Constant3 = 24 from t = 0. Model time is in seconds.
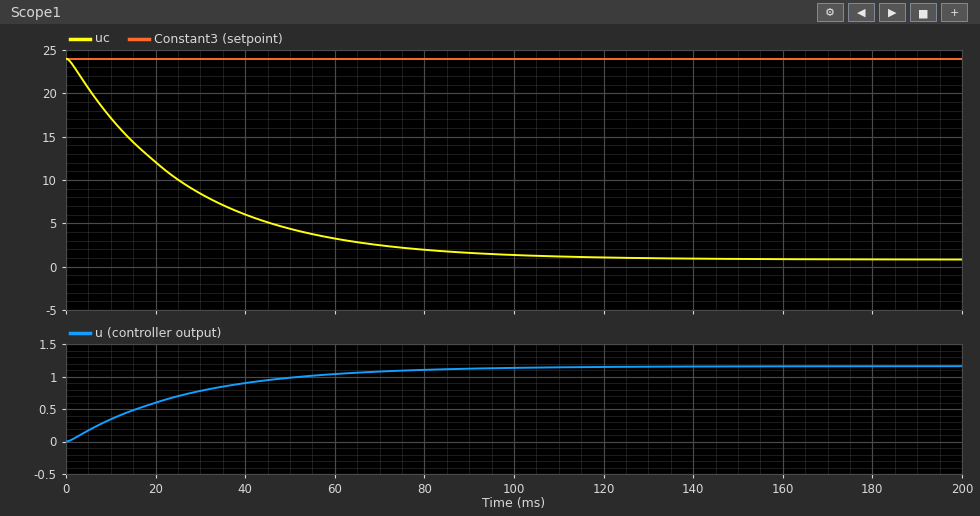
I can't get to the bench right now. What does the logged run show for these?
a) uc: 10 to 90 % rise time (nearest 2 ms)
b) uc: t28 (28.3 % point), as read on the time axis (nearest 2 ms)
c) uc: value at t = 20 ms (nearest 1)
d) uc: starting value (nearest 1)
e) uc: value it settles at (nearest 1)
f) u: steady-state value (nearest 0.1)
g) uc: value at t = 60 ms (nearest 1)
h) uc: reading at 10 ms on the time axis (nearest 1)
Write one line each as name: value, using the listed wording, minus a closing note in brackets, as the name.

uc: 10 to 90 % rise time: 58 ms
uc: t28 (28.3 % point), as read on the time axis: 10 ms
uc: value at t = 20 ms: 12
uc: starting value: 24
uc: value it settles at: 1
u: steady-state value: 1.2
uc: value at t = 60 ms: 3
uc: reading at 10 ms on the time axis: 17
